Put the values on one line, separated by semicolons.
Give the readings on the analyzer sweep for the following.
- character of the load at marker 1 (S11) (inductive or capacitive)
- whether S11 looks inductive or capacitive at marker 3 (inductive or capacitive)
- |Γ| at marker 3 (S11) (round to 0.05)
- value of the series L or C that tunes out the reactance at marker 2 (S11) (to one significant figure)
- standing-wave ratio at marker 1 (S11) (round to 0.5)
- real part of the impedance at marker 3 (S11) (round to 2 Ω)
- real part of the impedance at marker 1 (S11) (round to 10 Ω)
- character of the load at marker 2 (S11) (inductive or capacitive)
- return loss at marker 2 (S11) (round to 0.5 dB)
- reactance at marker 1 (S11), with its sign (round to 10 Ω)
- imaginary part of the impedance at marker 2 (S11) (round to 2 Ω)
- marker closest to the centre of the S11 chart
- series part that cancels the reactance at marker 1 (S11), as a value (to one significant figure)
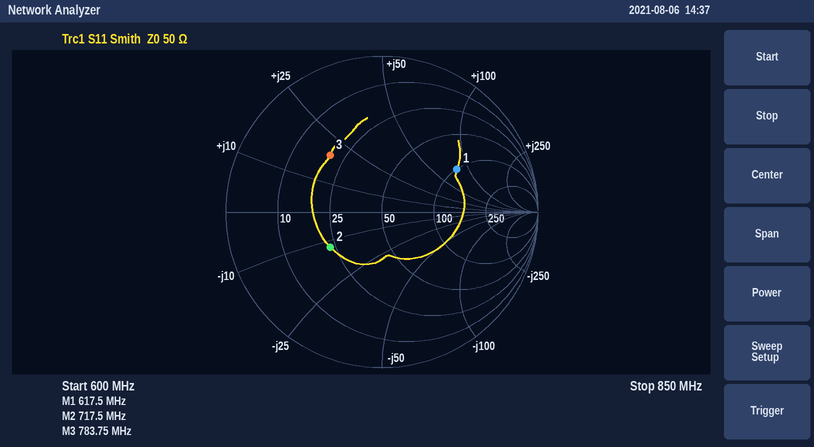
inductive; inductive; 0.50; 3 nH; 3.5; 20 Ω; 100 Ω; capacitive; 8.0 dB; +80 Ω; -12 Ω; marker 2; 3 pF
